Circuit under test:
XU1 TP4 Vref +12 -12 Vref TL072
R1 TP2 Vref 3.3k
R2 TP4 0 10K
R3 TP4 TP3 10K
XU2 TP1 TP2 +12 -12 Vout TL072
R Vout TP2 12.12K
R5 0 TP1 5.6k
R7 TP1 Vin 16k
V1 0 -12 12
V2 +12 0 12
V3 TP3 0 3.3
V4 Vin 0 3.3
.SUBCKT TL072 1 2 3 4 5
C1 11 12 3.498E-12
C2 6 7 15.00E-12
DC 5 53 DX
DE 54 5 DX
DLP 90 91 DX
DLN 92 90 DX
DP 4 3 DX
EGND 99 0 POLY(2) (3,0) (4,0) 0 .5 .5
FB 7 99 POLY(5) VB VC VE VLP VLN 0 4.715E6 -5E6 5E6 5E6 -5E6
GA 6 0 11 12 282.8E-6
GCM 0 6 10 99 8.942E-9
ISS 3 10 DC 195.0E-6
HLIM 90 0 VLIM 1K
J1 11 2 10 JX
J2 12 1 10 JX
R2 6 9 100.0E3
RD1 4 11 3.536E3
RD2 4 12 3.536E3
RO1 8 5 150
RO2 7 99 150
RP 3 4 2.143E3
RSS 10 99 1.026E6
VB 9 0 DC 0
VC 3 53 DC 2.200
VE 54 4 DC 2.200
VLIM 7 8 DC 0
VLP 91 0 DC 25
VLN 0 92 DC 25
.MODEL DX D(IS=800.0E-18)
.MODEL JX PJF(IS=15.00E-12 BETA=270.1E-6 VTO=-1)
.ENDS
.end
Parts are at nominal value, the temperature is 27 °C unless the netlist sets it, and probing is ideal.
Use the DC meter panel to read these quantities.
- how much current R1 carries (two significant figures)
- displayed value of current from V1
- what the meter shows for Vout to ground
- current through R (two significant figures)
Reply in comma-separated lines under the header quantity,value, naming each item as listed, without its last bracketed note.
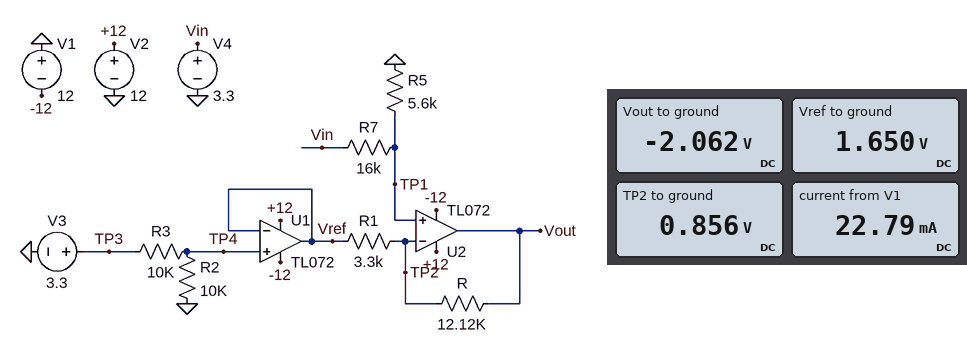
quantity,value
how much current R1 carries,240 µA
displayed value of current from V1,22.79 mA
what the meter shows for Vout to ground,-2.062 V
current through R,240 µA
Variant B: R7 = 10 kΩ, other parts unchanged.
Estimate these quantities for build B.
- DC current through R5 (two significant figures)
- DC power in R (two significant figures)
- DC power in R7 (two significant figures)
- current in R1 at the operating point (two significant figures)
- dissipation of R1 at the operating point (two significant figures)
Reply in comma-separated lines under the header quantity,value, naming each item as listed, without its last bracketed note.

quantity,value
DC current through R5,210 µA
DC power in R,240 µW
DC power in R7,450 µW
current in R1 at the operating point,140 µA
dissipation of R1 at the operating point,66 µW
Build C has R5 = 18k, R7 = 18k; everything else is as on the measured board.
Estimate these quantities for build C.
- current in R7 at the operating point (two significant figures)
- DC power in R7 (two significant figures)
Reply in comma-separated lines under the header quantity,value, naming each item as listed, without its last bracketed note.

quantity,value
current in R7 at the operating point,92 µA
DC power in R7,150 µW
